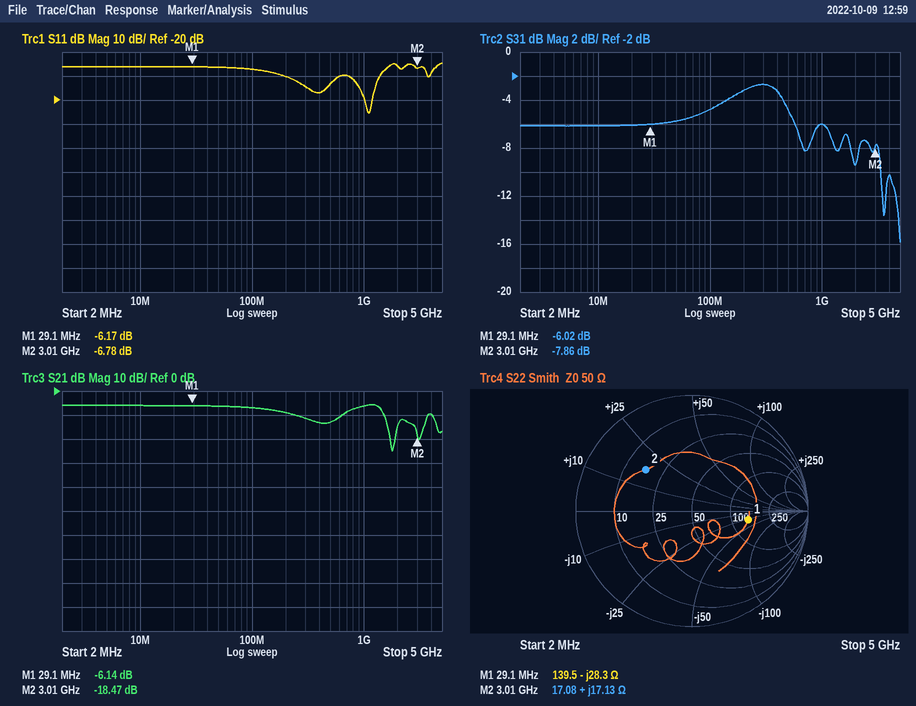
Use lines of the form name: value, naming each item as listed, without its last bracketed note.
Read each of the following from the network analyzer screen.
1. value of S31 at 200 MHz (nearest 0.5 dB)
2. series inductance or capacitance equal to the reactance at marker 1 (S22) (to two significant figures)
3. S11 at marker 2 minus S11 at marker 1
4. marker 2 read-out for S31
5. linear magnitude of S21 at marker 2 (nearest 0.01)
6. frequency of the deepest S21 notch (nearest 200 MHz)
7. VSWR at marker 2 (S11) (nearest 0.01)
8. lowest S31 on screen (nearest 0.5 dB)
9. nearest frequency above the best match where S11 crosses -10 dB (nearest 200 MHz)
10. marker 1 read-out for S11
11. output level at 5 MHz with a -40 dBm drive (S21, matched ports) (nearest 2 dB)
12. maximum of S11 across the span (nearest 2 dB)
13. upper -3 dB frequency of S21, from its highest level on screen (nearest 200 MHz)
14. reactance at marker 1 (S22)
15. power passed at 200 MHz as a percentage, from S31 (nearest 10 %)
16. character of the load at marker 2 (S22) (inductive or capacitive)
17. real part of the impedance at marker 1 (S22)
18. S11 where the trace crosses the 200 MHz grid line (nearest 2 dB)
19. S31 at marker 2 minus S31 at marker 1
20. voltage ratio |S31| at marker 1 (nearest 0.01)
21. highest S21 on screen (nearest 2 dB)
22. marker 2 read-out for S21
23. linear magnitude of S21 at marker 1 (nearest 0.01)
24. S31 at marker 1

value of S31 at 200 MHz: -3.0 dB
series inductance or capacitance equal to the reactance at marker 1 (S22): 190 pF
S11 at marker 2 minus S11 at marker 1: -0.61 dB
marker 2 read-out for S31: -7.86 dB
linear magnitude of S21 at marker 2: 0.12
frequency of the deepest S21 notch: 1.8 GHz
VSWR at marker 2 (S11): 2.69
lowest S31 on screen: -16.0 dB
nearest frequency above the best match where S11 crosses -10 dB: 1.4 GHz
marker 1 read-out for S11: -6.17 dB
output level at 5 MHz with a -40 dBm drive (S21, matched ports): -46 dBm
maximum of S11 across the span: -4 dB
upper -3 dB frequency of S21, from its highest level on screen: 1.4 GHz
reactance at marker 1: -28.3 Ω
power passed at 200 MHz as a percentage, from S31: 50 %
character of the load at marker 2 (S22): inductive
real part of the impedance at marker 1: 139.5 Ω
S11 where the trace crosses the 200 MHz grid line: -10 dB
S31 at marker 2 minus S31 at marker 1: -1.84 dB
voltage ratio |S31| at marker 1: 0.50
highest S21 on screen: -6 dB
marker 2 read-out for S21: -18.47 dB
linear magnitude of S21 at marker 1: 0.49
S31 at marker 1: -6.02 dB
